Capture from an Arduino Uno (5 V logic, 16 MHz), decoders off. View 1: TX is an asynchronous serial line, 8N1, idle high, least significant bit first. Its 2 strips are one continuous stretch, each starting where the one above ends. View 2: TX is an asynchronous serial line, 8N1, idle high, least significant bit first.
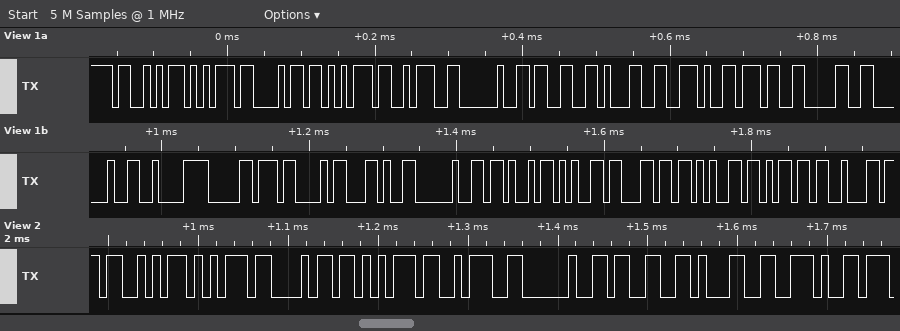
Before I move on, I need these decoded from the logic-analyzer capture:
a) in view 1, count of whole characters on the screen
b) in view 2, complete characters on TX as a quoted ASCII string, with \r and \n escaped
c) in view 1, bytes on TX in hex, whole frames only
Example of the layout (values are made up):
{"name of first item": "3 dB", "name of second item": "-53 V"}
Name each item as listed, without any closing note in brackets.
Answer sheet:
{"in view 1, count of whole characters on the screen": "23", "in view 2, complete characters on TX as a quoted ASCII string, with \\r and \\n escaped": "\"Suhu: 31.\"", "in view 1, bytes on TX in hex, whole frames only": "0x53 0x75 0x68 0x75 0x3A 0x20 0x33 0x31 0x2E 0x37 0x30 0x20 0xC2 0xB0 0x43 0x2C 0x20 0x4B 0x65 0x6C 0x65 0x6D 0x62"}
